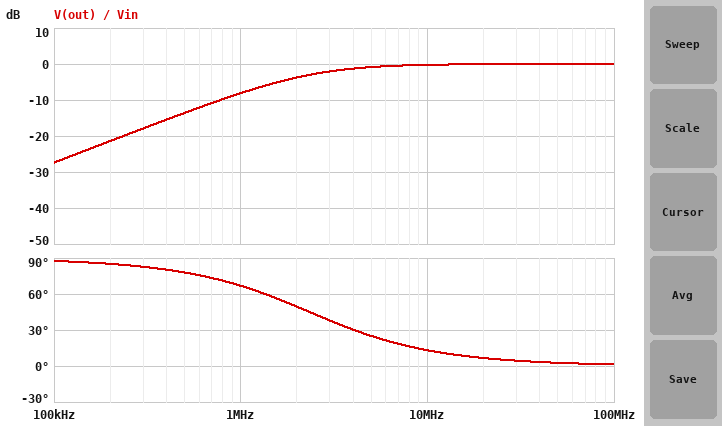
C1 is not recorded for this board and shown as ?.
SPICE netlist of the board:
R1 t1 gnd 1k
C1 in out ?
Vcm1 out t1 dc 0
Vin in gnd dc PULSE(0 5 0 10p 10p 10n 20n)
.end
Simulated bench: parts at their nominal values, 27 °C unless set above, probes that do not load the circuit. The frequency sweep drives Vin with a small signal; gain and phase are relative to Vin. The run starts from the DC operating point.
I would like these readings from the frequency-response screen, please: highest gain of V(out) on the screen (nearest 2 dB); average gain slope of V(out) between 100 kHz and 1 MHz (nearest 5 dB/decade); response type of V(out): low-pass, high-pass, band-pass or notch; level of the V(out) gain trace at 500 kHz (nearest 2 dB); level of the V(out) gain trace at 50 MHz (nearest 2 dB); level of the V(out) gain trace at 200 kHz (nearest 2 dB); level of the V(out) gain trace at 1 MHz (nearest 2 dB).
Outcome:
0 dB
20 dB/decade
high-pass
-14 dB
0 dB
-22 dB
-8 dB
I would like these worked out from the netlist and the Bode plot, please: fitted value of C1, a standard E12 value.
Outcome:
68 pF
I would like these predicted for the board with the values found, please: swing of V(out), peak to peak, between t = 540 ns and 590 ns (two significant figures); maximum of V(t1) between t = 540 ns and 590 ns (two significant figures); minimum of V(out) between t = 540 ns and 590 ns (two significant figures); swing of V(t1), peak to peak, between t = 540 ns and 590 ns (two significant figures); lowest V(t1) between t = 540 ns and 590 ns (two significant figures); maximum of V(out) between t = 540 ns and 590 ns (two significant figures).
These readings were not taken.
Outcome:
5.4 V
2.7 V
-2.7 V
5.4 V
-2.7 V
2.7 V
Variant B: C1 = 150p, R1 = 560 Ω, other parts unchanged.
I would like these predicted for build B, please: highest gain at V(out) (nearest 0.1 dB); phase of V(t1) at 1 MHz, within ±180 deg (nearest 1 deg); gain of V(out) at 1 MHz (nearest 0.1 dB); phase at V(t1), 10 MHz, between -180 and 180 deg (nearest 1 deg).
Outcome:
0 dB
62 deg
-6.6 dB
11 deg
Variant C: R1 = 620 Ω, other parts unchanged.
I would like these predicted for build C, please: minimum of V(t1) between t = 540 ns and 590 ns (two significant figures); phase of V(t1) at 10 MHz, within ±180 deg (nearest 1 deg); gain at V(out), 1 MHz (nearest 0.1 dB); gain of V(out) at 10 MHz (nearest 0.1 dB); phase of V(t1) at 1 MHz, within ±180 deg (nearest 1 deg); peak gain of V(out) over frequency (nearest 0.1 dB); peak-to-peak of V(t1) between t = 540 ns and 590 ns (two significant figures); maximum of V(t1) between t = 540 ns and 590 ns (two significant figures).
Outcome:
-2.8 V
21 deg
-11.8 dB
-0.6 dB
75 deg
0 dB
5.6 V
2.8 V
